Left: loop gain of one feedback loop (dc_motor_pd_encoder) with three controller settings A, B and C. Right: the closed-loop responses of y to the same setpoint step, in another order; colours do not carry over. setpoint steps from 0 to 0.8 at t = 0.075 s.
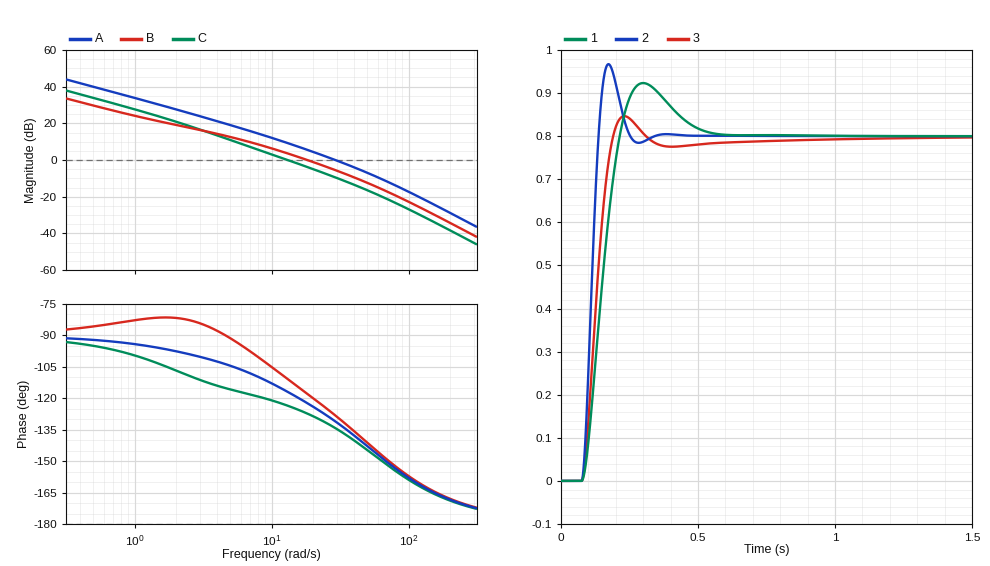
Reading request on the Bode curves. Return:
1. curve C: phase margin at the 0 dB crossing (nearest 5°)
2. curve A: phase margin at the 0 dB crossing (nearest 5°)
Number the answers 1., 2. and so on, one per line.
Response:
1. 55°
2. 50°
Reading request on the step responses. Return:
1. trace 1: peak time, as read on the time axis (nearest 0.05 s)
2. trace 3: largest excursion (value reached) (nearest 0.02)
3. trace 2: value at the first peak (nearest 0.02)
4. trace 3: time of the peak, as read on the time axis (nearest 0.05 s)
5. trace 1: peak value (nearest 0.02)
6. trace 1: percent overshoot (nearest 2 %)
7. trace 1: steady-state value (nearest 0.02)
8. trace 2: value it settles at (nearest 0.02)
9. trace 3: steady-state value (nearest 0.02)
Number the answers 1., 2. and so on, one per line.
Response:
1. 0.30 s
2. 0.84
3. 0.96
4. 0.25 s
5. 0.92
6. 16 %
7. 0.80
8. 0.80
9. 0.80
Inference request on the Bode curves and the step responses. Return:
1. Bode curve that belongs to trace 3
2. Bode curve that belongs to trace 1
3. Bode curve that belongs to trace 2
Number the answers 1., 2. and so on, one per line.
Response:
1. B
2. C
3. A
